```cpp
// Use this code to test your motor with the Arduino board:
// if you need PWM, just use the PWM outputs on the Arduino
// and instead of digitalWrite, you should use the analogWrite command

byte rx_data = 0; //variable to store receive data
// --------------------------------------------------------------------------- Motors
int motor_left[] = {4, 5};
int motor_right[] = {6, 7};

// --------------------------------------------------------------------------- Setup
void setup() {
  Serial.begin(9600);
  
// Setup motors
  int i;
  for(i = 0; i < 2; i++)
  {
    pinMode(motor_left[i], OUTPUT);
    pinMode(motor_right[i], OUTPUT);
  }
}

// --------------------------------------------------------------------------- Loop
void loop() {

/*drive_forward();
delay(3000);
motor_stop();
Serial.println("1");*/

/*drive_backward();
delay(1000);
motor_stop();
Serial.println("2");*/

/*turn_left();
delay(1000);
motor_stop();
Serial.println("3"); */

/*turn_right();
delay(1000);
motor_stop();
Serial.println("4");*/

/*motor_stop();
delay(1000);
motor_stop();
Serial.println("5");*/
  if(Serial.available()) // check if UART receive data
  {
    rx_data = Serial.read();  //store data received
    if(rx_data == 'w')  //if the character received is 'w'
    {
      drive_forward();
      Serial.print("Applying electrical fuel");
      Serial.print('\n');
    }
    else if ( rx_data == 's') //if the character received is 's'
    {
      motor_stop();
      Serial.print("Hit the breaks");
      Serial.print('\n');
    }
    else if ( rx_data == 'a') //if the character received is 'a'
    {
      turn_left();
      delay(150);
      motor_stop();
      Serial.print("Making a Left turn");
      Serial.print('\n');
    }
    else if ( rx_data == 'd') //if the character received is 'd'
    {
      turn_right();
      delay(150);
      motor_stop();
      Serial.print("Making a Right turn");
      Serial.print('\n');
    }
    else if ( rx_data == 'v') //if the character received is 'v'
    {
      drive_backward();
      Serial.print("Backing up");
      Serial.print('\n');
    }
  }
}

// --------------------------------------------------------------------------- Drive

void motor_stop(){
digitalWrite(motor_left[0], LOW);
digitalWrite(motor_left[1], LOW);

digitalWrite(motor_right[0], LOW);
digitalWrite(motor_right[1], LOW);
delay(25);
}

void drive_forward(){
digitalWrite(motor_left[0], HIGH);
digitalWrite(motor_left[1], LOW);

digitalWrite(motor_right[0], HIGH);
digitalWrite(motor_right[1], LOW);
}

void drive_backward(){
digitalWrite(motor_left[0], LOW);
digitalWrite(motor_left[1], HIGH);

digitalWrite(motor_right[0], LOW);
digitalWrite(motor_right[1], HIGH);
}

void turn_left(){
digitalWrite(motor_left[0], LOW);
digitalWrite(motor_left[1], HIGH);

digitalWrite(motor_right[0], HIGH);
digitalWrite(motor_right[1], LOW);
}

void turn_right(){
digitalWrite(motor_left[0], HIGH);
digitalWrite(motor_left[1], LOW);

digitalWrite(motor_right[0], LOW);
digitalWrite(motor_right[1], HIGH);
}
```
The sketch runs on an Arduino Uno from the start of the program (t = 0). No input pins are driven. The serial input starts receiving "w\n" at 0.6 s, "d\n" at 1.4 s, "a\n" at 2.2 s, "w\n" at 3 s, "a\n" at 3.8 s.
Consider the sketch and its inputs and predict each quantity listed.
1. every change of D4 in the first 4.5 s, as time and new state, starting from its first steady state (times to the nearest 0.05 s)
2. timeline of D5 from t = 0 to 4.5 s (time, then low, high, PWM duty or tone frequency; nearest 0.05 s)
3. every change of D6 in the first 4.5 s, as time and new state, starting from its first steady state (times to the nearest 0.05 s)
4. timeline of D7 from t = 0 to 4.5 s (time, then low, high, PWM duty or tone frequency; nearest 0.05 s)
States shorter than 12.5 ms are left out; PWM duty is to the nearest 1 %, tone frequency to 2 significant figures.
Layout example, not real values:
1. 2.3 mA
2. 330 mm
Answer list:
1. 0 s low; 0.6 s high; 1.55 s low; 3 s high; 3.8 s low
2. 0 s low; 2.2 s high; 2.35 s low; 3.8 s high; 3.95 s low
3. 0 s low; 0.6 s high; 1.4 s low; 2.2 s high; 2.35 s low; 3 s high; 3.95 s low
4. 0 s low; 1.4 s high; 1.55 s low
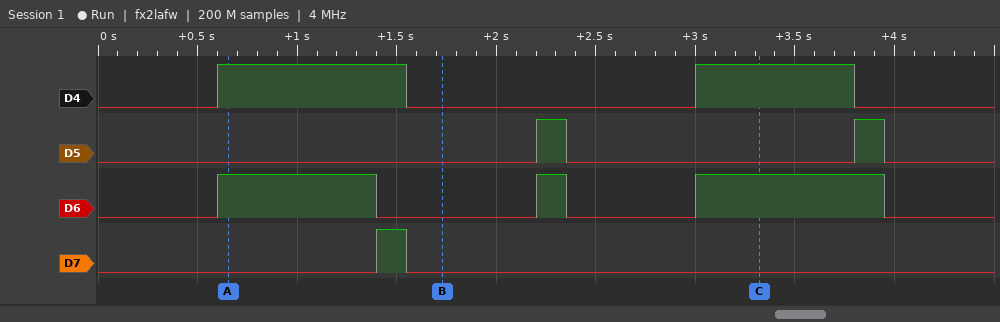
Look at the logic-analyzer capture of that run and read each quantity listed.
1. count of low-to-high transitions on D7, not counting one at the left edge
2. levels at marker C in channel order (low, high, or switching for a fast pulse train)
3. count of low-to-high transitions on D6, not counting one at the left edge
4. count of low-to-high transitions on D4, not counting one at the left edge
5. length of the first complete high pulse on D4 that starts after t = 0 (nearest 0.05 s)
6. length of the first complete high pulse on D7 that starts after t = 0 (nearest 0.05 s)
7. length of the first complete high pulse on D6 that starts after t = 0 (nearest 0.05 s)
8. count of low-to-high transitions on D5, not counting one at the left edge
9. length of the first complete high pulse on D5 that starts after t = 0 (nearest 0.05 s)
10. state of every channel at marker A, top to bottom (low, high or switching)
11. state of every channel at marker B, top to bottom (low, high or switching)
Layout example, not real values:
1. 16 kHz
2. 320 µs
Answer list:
1. 1
2. D4 high, D5 low, D6 high, D7 low
3. 3
4. 2
5. 0.95 s
6. 0.15 s
7. 0.80 s
8. 2
9. 0.15 s
10. D4 high, D5 low, D6 high, D7 low
11. D4 low, D5 low, D6 low, D7 low
